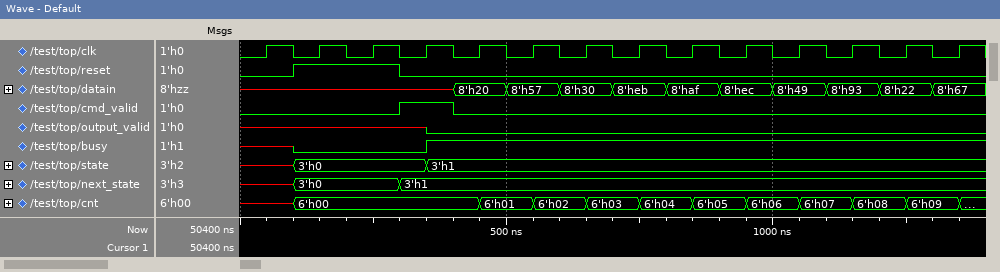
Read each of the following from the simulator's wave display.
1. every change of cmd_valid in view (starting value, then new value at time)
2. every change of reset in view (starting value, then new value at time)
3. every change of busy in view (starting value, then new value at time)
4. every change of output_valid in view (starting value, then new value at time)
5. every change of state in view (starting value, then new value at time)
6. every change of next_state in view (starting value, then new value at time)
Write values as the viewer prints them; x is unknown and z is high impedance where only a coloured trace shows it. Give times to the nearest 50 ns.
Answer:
0, 1 at 300 ns, 0 at 400 ns
0, 1 at 100 ns, 0 at 300 ns
x, 0 at 100 ns, 1 at 350 ns
x, 0 at 350 ns
x, 3'h0 at 100 ns, 3'h1 at 350 ns
x, 3'h0 at 100 ns, 3'h1 at 300 ns
